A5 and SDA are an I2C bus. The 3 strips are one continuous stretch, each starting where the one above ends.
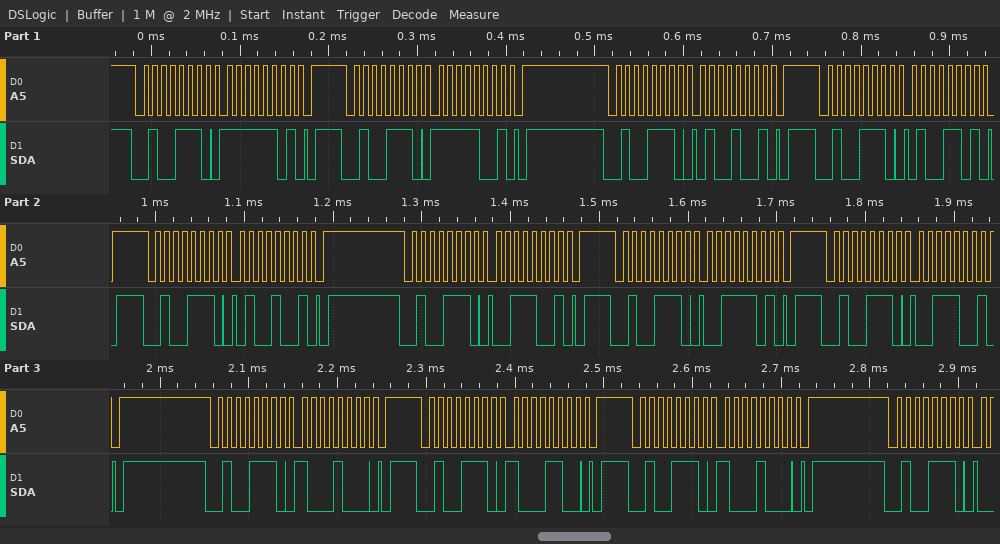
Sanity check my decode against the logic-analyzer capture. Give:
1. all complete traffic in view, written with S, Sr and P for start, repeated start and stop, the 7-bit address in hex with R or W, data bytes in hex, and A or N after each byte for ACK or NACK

S 27W A FD A P S 27W A F9 A P S 27W A 49 A P S 27W A 4D A P S 27W A 49 A P S 27W A 39 A P S 27W A 3D A P S 27W A 39 A P S 27W A 88 A P S 27W A 8C A P S 27W A 88 A P S 27W A
